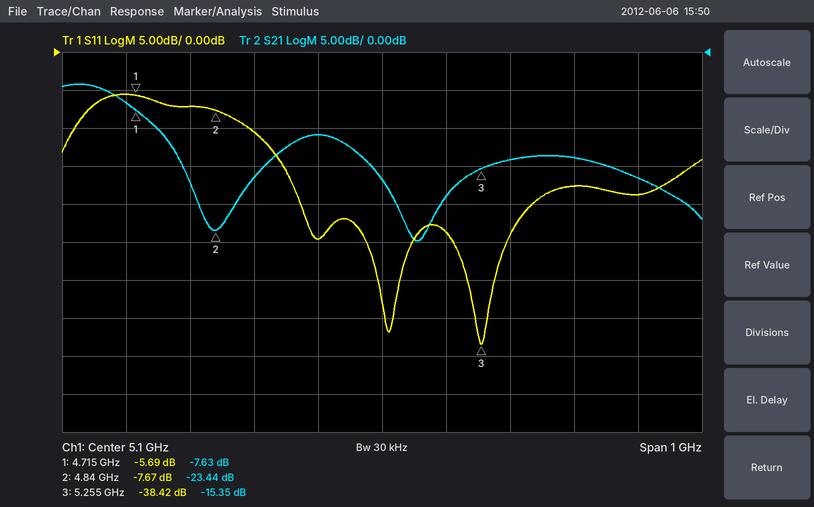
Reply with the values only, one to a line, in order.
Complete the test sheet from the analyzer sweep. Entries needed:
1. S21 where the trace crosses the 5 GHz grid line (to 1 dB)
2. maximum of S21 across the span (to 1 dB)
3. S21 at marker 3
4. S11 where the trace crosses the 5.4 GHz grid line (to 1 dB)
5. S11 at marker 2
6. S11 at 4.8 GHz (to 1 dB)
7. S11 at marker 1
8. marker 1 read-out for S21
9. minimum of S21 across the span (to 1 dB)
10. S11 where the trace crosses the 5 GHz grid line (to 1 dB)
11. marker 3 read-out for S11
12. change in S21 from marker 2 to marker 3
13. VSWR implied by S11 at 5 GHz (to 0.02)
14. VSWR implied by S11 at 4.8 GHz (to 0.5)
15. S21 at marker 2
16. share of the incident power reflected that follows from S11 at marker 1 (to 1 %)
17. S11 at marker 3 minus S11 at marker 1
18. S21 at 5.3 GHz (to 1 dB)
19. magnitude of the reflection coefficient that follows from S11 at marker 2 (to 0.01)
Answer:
-11 dB
-4 dB
-15.35 dB
-18 dB
-7.67 dB
-7 dB
-5.69 dB
-7.63 dB
-25 dB
-25 dB
-38.42 dB
8.09 dB
1.12
2.5
-23.44 dB
27 %
-32.73 dB
-14 dB
0.41
